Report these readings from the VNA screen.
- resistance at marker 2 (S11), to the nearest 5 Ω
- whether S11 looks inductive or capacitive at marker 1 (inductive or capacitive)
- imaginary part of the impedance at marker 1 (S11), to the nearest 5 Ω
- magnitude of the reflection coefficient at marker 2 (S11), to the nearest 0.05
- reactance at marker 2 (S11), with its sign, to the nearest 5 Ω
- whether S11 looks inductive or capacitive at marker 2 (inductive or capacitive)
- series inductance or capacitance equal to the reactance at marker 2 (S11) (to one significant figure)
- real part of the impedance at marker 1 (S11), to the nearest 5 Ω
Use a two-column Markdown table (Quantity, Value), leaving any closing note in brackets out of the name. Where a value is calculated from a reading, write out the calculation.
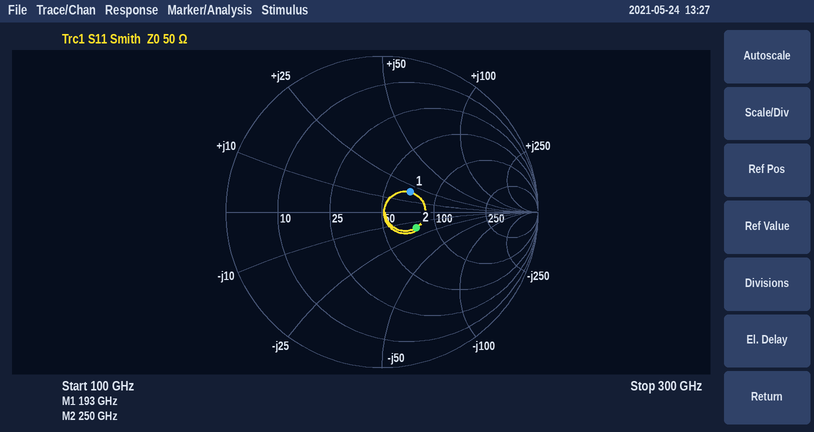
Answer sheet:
| Quantity | Value |
|---|---|
| resistance at marker 2 (S11), to the nearest 5 Ω | 75 Ω |
| whether S11 looks inductive or capacitive at marker 1 | inductive |
| imaginary part of the impedance at marker 1 (S11), to the nearest 5 Ω | +20 Ω |
| magnitude of the reflection coefficient at marker 2 (S11), to the nearest 0.05 | 0.25 |
| reactance at marker 2 (S11), with its sign, to the nearest 5 Ω | -15 Ω |
| whether S11 looks inductive or capacitive at marker 2 | capacitive |
| series inductance or capacitance equal to the reactance at marker 2 (S11) | C = 1/(2π × 250 GHz × 15 Ω) ≈ 42.4 fF, so 40 fF to one significant figure |
| real part of the impedance at marker 1 (S11), to the nearest 5 Ω | 70 Ω |
